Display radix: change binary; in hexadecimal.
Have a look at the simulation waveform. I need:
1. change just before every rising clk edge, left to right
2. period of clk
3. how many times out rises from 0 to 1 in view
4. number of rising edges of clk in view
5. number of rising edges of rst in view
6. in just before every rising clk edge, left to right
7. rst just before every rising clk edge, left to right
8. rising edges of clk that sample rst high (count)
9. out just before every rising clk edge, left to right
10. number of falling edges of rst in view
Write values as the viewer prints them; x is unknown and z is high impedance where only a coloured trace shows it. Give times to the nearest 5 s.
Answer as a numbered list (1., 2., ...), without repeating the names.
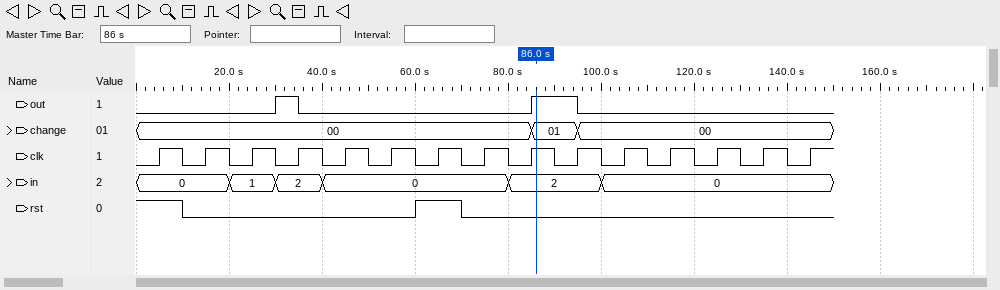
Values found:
1. 00, 00, 00, 00, 00, 00, 00, 00, 00, 01, 00, 00, 00, 00, 00
2. 10 s
3. 2
4. 15
5. 1
6. 0, 0, 1, 2, 0, 0, 0, 0, 2, 2, 0, 0, 0, 0, 0
7. 1 0 0 0 0 0 1 0 0 0 0 0 0 0 0
8. 2
9. 0 0 0 1 0 0 0 0 0 1 0 0 0 0 0
10. 2
